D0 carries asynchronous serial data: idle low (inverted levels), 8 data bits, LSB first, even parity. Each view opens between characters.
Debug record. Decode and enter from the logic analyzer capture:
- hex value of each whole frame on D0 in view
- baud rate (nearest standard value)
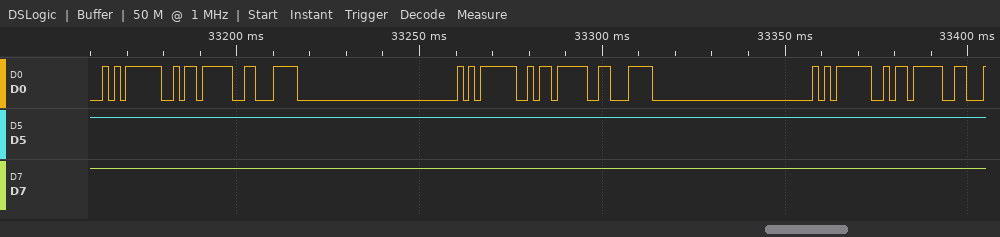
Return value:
05, 09, 0E, 05, 09, 0E, 05, 09
600 baud
